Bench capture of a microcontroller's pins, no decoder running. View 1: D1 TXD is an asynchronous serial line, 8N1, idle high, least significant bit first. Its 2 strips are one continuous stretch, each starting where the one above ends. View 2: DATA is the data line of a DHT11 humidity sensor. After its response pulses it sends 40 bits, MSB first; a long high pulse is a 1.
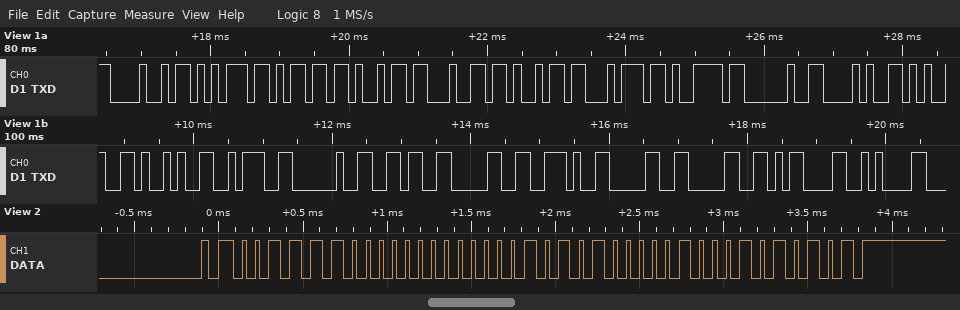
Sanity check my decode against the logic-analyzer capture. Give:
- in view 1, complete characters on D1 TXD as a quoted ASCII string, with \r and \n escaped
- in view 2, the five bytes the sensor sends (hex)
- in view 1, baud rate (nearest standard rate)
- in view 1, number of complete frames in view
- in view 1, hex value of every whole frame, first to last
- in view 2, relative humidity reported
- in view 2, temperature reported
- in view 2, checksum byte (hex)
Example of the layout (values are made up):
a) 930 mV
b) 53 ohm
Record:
a) "Humidity (%): 60.00\r\n"
b) 3C 00 15 04 55
c) 9600 baud
d) 21
e) 48 75 6D 69 64 69 74 79 20 28 25 29 3A 20 36 30 2E 30 30 0D 0A
f) 60 %
g) 21.4 °C
h) 0x55
